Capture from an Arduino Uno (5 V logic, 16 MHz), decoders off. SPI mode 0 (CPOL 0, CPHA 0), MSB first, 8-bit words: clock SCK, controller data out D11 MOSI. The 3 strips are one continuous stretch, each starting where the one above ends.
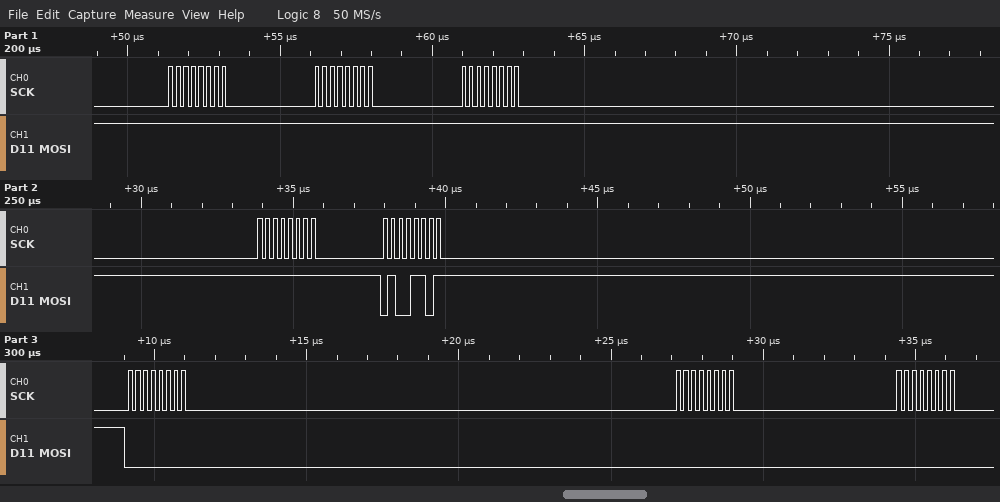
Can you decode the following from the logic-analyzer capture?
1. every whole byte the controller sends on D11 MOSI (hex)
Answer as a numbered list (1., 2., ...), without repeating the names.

1. FF FF FF FF 4D 00 00 00
